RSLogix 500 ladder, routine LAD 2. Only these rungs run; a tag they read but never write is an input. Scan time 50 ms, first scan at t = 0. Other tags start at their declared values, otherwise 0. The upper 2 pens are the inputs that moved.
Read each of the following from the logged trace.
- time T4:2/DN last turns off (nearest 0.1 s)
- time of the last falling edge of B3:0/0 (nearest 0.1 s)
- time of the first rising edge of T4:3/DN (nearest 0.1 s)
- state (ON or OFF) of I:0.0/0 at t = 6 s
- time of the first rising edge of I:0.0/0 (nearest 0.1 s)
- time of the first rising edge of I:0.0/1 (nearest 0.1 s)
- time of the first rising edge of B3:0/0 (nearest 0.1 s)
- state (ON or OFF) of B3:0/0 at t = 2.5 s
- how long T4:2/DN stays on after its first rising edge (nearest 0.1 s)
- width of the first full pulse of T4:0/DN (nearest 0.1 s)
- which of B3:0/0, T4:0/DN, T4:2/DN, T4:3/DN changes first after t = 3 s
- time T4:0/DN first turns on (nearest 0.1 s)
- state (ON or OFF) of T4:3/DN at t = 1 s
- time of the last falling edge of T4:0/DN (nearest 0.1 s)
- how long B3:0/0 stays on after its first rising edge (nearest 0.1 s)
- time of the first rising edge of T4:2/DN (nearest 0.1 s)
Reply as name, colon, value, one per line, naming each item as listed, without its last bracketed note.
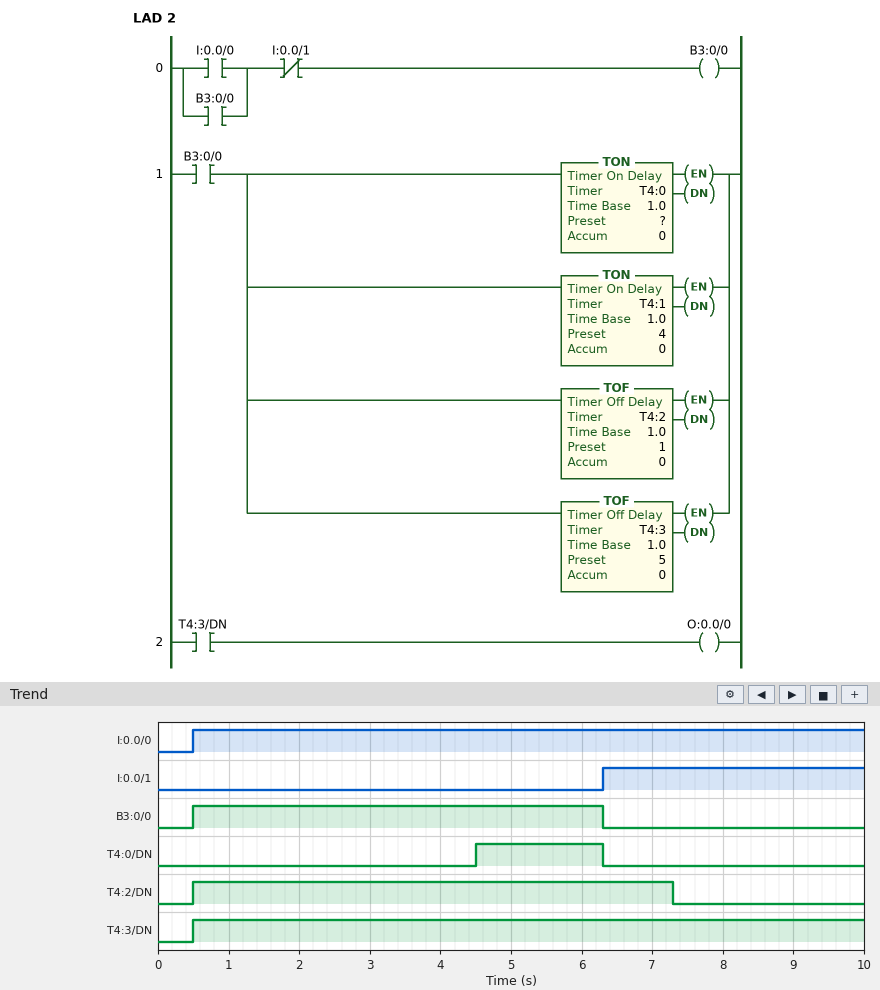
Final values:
time T4:2/DN last turns off: 7.3 s
time of the last falling edge of B3:0/0: 6.3 s
time of the first rising edge of T4:3/DN: 0.5 s
state (ON or OFF) of I:0.0/0 at t = 6 s: ON
time of the first rising edge of I:0.0/0: 0.5 s
time of the first rising edge of I:0.0/1: 6.3 s
time of the first rising edge of B3:0/0: 0.5 s
state (ON or OFF) of B3:0/0 at t = 2.5 s: ON
how long T4:2/DN stays on after its first rising edge: 6.8 s
width of the first full pulse of T4:0/DN: 1.8 s
which of B3:0/0, T4:0/DN, T4:2/DN, T4:3/DN changes first after t = 3 s: T4:0/DN
time T4:0/DN first turns on: 4.5 s
state (ON or OFF) of T4:3/DN at t = 1 s: ON
time of the last falling edge of T4:0/DN: 6.3 s
how long B3:0/0 stays on after its first rising edge: 5.8 s
time of the first rising edge of T4:2/DN: 0.5 s
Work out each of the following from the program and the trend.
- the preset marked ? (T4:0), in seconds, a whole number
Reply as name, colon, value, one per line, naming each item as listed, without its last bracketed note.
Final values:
the preset marked ? (T4:0), in seconds, a whole number: 4 s
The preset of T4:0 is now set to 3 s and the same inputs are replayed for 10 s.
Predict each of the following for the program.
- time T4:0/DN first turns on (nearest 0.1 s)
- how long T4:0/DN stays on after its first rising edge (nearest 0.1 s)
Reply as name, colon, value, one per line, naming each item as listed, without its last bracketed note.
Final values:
time T4:0/DN first turns on: 3.5 s
how long T4:0/DN stays on after its first rising edge: 2.8 s
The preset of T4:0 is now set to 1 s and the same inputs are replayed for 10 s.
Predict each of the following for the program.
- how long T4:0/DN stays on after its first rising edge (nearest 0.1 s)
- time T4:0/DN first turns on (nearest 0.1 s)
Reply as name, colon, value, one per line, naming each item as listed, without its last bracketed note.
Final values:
how long T4:0/DN stays on after its first rising edge: 4.8 s
time T4:0/DN first turns on: 1.5 s
